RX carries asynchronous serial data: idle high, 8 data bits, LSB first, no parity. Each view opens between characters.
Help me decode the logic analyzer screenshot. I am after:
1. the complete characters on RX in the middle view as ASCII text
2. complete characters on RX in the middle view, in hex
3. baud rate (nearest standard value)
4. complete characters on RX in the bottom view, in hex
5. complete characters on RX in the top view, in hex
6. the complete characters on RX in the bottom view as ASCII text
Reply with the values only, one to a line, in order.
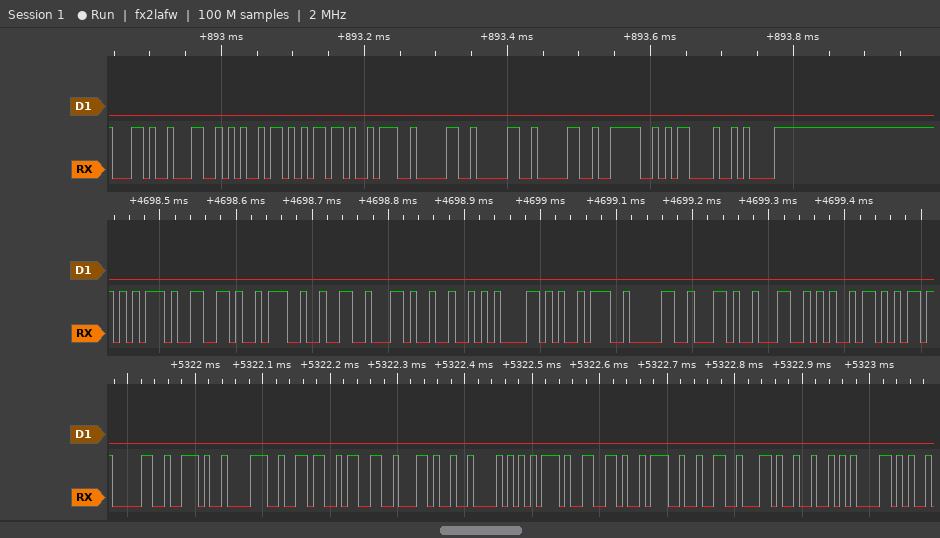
"uf:2,RX:0,Li"
75, 66, 3A, 32, 2C, 52, 58, 3A, 30, 2C, 4C, 69
115200 baud
30, 2E, 38, 36, 33, 2C, 42, 75, 66, 3A, 32, 2C, 52, 58
2C, 4C, 69, 6D, 3A, 30, 30, 30, 3E, 0D, 0A
"0.863,Buf:2,RX"
